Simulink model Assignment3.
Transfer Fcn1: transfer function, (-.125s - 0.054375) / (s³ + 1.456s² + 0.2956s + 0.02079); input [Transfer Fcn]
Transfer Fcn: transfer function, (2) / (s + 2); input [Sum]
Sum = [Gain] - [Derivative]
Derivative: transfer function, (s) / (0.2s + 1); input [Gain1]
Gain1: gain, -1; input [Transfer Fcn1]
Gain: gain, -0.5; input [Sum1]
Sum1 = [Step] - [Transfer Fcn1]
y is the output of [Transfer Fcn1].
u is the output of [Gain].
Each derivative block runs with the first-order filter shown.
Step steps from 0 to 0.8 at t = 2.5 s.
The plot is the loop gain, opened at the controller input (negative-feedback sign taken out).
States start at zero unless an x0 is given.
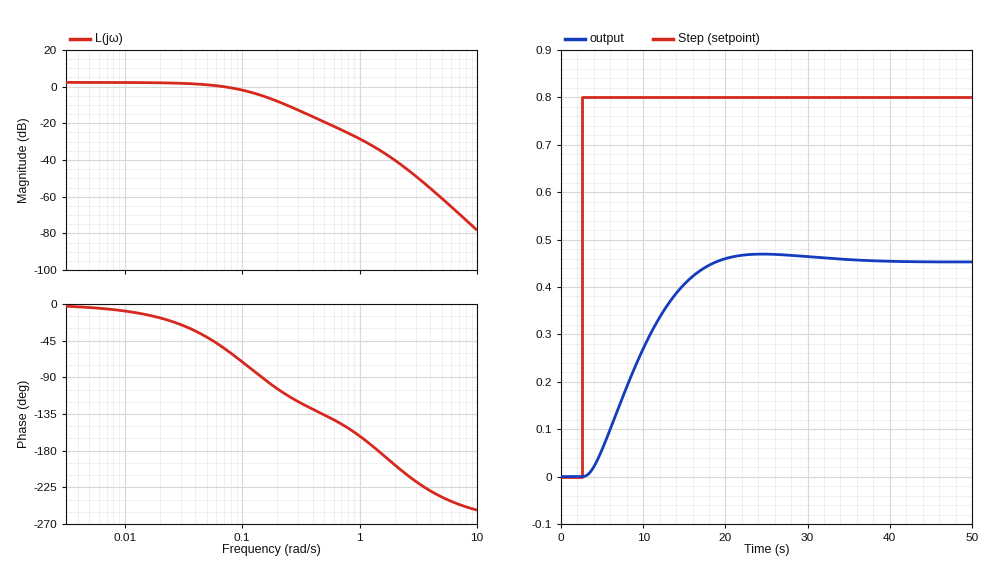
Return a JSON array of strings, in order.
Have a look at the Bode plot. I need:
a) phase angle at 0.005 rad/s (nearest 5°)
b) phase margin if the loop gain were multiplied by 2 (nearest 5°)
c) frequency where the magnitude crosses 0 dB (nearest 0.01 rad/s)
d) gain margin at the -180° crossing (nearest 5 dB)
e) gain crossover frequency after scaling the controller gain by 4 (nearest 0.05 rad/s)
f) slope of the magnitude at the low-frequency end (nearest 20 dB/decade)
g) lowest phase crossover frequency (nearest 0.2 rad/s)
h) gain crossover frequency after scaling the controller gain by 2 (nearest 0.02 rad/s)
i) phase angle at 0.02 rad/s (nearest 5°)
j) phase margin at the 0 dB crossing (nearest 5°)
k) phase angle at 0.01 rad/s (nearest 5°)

["-5°", "85°", "0.07 rad/s", "35 dB", "0.30 rad/s", "0 dB/decade", "1.4 rad/s", "0.16 rad/s", "-15°", "125°", "-10°"]
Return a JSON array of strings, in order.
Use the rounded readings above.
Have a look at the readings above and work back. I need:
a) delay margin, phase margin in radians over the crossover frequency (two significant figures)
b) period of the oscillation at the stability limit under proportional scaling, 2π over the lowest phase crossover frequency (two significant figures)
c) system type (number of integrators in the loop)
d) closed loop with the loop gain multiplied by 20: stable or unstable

["31 s", "4.5 s", "0", "stable"]
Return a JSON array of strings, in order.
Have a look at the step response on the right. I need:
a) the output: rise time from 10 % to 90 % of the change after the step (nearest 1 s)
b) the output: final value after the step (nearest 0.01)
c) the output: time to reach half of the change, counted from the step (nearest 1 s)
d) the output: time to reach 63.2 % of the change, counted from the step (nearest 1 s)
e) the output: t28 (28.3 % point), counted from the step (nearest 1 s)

["10 s", "0.45", "6 s", "8 s", "4 s"]
